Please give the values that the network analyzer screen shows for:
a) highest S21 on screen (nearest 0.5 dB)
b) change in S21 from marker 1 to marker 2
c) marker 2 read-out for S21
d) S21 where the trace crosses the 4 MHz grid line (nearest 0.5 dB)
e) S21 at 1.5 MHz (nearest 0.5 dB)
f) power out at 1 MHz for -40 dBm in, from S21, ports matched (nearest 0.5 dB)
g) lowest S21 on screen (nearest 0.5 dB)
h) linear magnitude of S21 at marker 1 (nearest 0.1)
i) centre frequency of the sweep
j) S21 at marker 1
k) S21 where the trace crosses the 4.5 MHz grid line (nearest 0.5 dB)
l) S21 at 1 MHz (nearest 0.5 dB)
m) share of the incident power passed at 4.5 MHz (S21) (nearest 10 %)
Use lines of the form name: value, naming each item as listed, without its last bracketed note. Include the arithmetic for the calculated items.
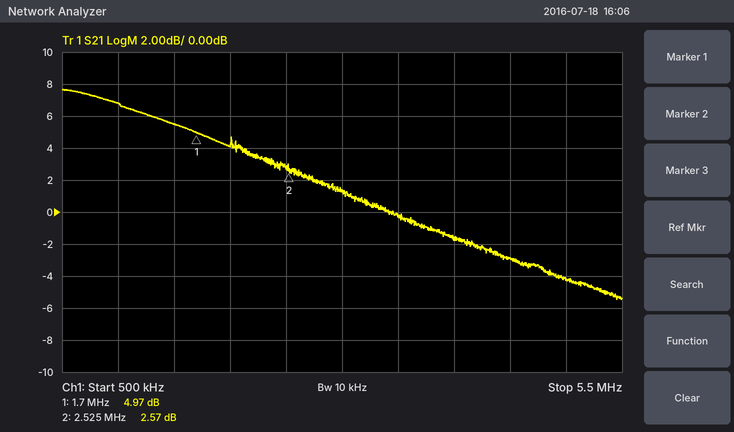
highest S21 on screen: 7.5 dB
change in S21 from marker 1 to marker 2: 2.57 − (4.97) = -2.40 dB
marker 2 read-out for S21: 2.57 dB
S21 where the trace crosses the 4 MHz grid line: -1.5 dB
S21 at 1.5 MHz: 5.5 dB
power out at 1 MHz for -40 dBm in, from S21, ports matched: -40 dBm + (7.0 dB) = -33.0 dBm
lowest S21 on screen: -5.5 dB
linear magnitude of S21 at marker 1: 10^(4.97/20) ≈ 1.8
centre frequency of the sweep: 3 MHz
S21 at marker 1: 4.97 dB
S21 where the trace crosses the 4.5 MHz grid line: -3.0 dB
S21 at 1 MHz: 7.0 dB
share of the incident power passed at 4.5 MHz (S21): 10^(-3/10) ≈ 50 %
